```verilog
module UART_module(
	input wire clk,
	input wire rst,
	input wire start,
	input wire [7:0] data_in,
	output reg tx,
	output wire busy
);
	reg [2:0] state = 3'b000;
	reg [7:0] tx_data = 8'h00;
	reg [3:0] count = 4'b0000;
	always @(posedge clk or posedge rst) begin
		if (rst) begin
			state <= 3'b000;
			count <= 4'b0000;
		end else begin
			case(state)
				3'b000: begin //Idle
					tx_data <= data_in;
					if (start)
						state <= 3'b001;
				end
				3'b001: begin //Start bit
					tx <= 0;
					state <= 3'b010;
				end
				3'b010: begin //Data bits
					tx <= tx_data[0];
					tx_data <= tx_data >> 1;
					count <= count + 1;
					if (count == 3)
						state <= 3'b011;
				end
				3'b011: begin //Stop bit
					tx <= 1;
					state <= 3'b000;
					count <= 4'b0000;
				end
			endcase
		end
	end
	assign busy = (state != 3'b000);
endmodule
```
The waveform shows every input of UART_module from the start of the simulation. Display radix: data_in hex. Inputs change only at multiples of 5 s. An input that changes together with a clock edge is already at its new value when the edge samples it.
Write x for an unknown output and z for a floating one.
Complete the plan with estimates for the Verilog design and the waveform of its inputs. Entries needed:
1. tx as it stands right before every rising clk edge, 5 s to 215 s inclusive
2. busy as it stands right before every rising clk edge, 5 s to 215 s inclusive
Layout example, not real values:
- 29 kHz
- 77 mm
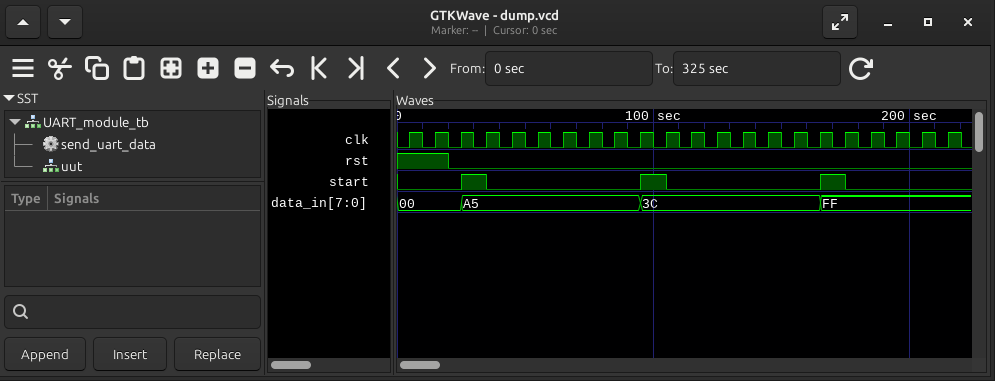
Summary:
- x x x x 0 1 0 1 0 1 1 0 0 0 1 1 1 1 0 1 1 1
- 0 0 0 1 1 1 1 1 1 0 1 1 1 1 1 1 0 1 1 1 1 1
